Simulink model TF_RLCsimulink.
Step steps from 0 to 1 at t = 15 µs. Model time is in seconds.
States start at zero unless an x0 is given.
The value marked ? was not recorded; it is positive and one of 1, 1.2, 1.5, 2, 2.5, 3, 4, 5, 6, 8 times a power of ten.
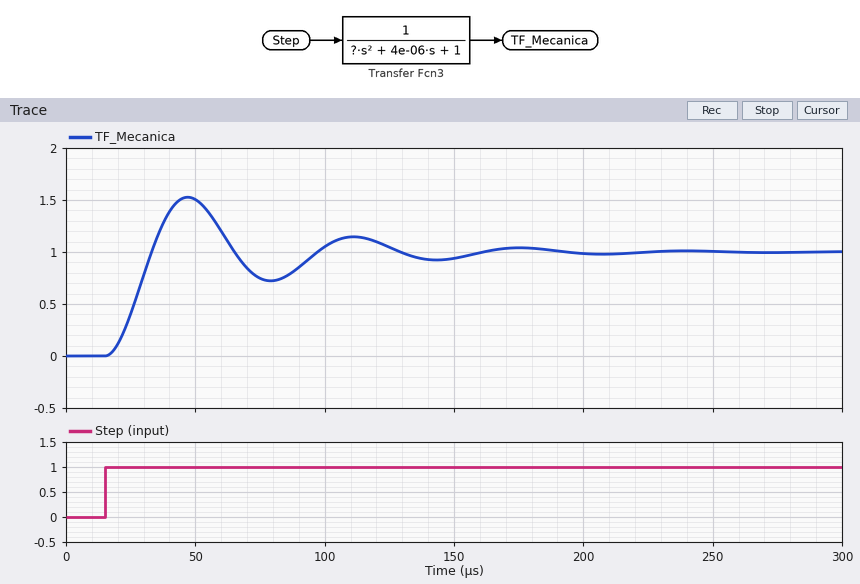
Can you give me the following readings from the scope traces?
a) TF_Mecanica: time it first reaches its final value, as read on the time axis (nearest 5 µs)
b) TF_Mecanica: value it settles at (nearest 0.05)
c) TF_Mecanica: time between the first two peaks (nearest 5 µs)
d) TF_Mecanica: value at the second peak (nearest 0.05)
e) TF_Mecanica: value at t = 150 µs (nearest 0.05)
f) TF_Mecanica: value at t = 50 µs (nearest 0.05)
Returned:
35 µs
1.00
65 µs
1.15
0.95
1.50
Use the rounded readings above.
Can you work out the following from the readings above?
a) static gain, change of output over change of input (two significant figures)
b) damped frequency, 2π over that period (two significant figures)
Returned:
1.0
0.097 rad/µs
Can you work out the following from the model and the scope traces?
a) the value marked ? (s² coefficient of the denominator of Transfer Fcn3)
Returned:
1e-10
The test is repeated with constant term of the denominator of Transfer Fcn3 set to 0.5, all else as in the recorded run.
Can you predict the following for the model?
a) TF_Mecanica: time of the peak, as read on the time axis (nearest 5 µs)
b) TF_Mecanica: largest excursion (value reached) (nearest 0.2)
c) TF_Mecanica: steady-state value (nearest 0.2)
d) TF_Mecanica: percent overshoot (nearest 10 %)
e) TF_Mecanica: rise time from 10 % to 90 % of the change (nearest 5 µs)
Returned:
60 µs
2.8
2.0
40 %
20 µs
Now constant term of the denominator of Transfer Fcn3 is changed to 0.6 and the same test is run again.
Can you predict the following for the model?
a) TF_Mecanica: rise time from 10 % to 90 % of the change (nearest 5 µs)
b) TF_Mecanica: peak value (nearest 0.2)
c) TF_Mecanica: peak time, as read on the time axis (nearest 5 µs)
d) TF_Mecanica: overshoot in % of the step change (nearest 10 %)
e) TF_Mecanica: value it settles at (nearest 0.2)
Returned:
15 µs
2.4
55 µs
40 %
1.6
